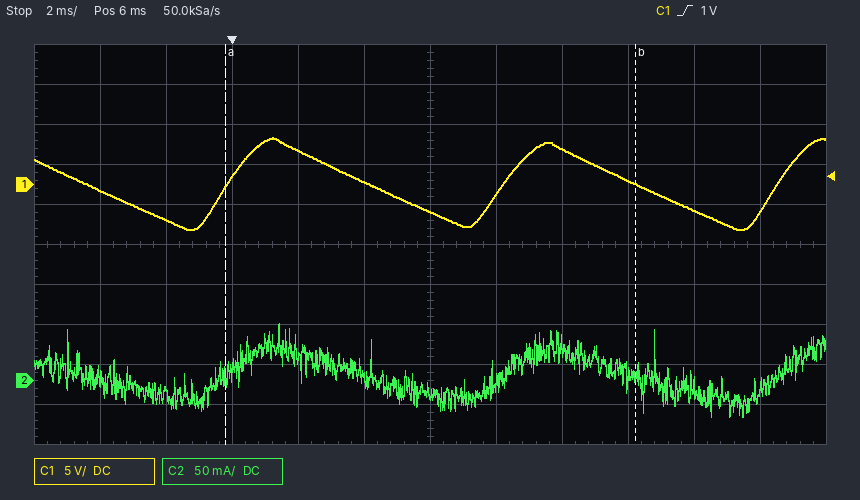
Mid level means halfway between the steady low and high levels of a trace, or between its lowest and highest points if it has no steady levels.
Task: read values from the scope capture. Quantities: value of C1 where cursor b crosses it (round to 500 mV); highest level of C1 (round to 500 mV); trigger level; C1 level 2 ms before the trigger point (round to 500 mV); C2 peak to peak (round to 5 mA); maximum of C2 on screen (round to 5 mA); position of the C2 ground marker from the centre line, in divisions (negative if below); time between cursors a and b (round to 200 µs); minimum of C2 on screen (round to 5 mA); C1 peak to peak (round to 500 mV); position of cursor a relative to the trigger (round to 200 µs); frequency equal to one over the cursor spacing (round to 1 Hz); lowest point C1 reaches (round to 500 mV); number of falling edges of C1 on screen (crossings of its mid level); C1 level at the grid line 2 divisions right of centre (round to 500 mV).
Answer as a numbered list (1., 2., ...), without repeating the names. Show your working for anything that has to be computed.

1. 0.0 V
2. 6.0 V
3. 1 V
4. -4.5 V
5. 70 mA − (-45 mA) = 115 mA
6. 70 mA
7. -3.4 div
8. 12.4 ms
9. -45 mA
10. 6.0 V − (-5.5 V) = 11.5 V
11. -200 µs
12. 1 / 12.4 ms ≈ 81 Hz
13. -5.5 V
14. 3
15. 4.5 V
